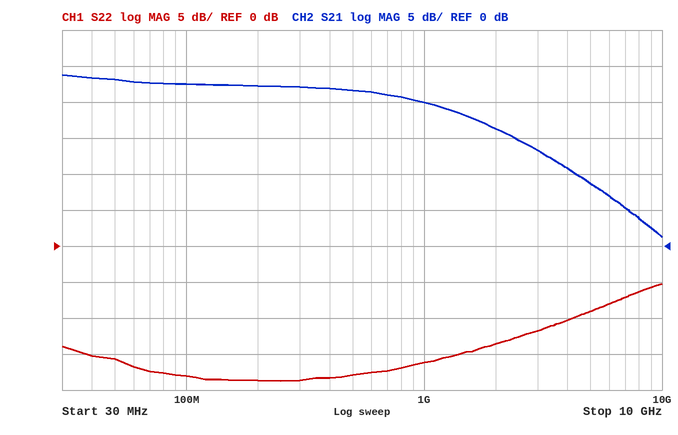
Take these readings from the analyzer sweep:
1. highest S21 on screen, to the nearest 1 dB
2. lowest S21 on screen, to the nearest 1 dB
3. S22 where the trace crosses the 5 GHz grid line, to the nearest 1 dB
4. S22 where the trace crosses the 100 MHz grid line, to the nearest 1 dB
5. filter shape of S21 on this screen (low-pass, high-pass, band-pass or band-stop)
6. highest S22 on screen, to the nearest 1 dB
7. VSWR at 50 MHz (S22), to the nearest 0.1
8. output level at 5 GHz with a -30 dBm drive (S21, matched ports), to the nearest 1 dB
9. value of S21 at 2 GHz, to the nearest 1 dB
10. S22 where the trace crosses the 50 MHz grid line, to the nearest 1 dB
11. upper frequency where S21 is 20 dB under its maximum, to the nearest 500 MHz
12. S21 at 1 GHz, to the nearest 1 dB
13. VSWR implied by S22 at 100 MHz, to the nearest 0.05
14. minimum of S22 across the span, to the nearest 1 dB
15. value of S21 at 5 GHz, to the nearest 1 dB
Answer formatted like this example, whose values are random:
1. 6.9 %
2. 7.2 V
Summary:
1. 24 dB
2. 1 dB
3. -9 dB
4. -18 dB
5. low-pass
6. -5 dB
7. 1.4
8. -21 dBm
9. 16 dB
10. -16 dB
11. 8.0 GHz
12. 20 dB
13. 1.30
14. -19 dB
15. 9 dB
